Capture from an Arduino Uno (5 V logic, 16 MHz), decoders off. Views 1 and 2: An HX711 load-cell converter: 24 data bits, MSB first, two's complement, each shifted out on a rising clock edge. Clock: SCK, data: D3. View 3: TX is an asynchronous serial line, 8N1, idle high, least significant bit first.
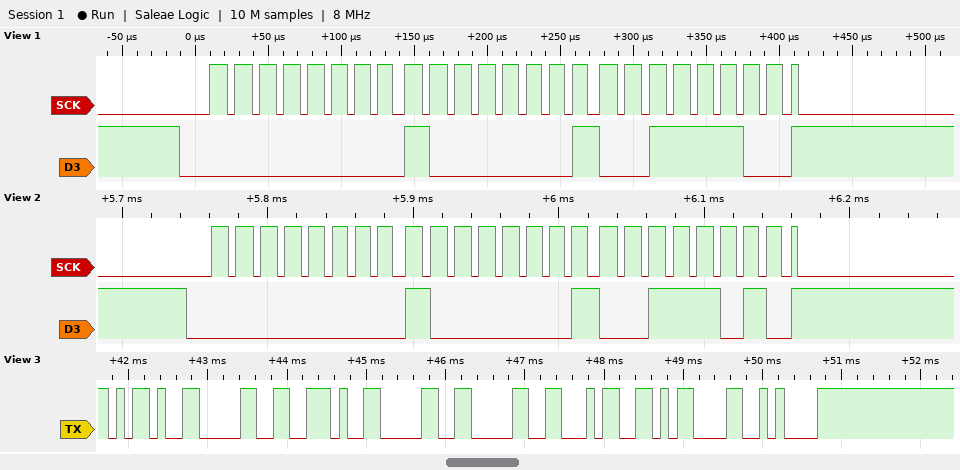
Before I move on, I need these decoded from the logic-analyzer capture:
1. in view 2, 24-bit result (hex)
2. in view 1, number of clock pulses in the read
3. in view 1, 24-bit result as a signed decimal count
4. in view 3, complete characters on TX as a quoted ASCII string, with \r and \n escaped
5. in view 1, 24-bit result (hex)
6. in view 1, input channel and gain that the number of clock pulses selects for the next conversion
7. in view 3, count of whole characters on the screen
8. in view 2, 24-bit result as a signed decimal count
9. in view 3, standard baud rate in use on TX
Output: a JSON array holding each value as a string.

["0x00813A", "25", "33084", "\"-0.004\\r\\n\"", "0x00813C", "channel A, gain 128", "8", "33082", "9600 baud"]
